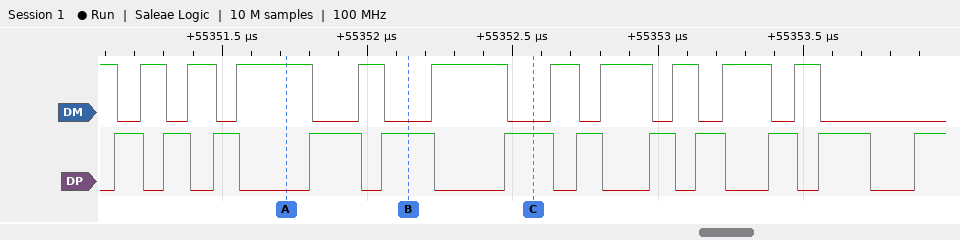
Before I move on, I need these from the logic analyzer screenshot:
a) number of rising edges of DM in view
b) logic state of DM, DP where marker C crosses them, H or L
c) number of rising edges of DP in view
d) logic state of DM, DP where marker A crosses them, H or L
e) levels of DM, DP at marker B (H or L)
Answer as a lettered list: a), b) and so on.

a) 10
b) DM=L, DP=H
c) 12
d) DM=H, DP=L
e) DM=L, DP=H
